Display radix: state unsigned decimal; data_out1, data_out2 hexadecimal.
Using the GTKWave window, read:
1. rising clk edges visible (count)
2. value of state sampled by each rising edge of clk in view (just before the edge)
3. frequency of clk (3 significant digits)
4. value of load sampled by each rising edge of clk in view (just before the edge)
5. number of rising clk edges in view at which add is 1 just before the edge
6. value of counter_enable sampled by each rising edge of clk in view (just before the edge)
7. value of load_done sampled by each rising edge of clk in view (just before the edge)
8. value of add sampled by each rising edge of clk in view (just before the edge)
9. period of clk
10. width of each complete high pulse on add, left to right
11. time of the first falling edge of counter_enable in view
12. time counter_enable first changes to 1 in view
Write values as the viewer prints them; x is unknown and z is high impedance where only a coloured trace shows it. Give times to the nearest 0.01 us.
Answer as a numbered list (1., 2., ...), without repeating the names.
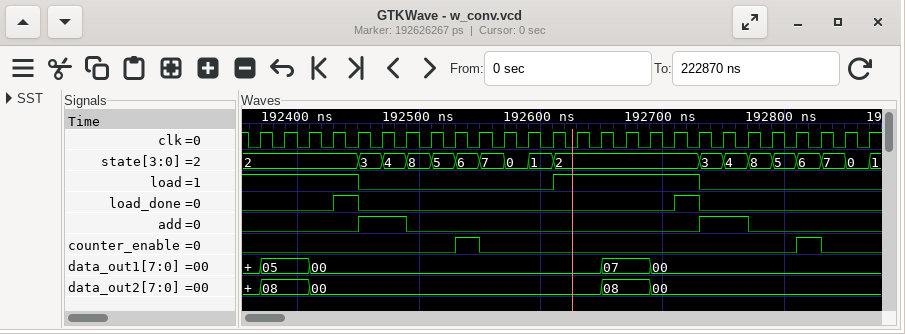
1. 26
2. 2, 2, 2, 2, 2, 3, 4, 8, 5, 6, 7, 0, 1, 2, 2, 2, 2, 2, 2, 3, 4, 8, 5, 6, 7, 0
3. 50.0 MHz
4. 1 1 1 1 1 0 0 0 0 0 0 0 0 1 1 1 1 1 1 0 0 0 0 0 0 0
5. 4
6. 0 0 0 0 0 0 0 0 0 1 0 0 0 0 0 0 0 0 0 0 0 0 0 1 0 0
7. 0 0 0 0 1 0 0 0 0 0 0 0 0 0 0 0 0 0 1 0 0 0 0 0 0 0
8. 0 0 0 0 0 1 1 0 0 0 0 0 0 0 0 0 0 0 0 1 1 0 0 0 0 0
9. 0.02 us
10. 0.04 us, 0.04 us
11. 192.55 us
12. 192.53 us
